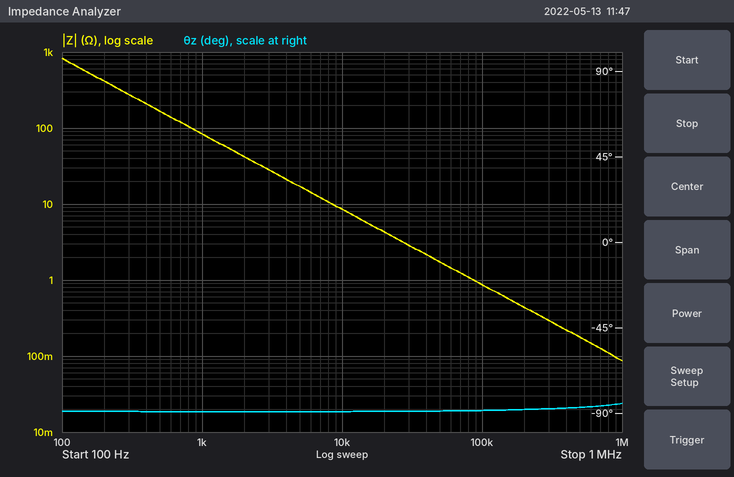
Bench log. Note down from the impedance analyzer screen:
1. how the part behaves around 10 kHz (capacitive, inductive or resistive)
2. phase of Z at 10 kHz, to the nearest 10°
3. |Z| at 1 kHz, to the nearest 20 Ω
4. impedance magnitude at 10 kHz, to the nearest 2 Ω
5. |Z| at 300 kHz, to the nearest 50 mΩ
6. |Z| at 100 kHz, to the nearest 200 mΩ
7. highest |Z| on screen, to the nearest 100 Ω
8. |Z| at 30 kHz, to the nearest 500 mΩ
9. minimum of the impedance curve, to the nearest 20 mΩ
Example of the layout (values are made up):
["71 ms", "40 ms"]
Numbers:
["capacitive", "-90°", "80 Ω", "8 Ω", "300 mΩ", "800 mΩ", "800 Ω", "3.0 Ω", "80 mΩ"]
